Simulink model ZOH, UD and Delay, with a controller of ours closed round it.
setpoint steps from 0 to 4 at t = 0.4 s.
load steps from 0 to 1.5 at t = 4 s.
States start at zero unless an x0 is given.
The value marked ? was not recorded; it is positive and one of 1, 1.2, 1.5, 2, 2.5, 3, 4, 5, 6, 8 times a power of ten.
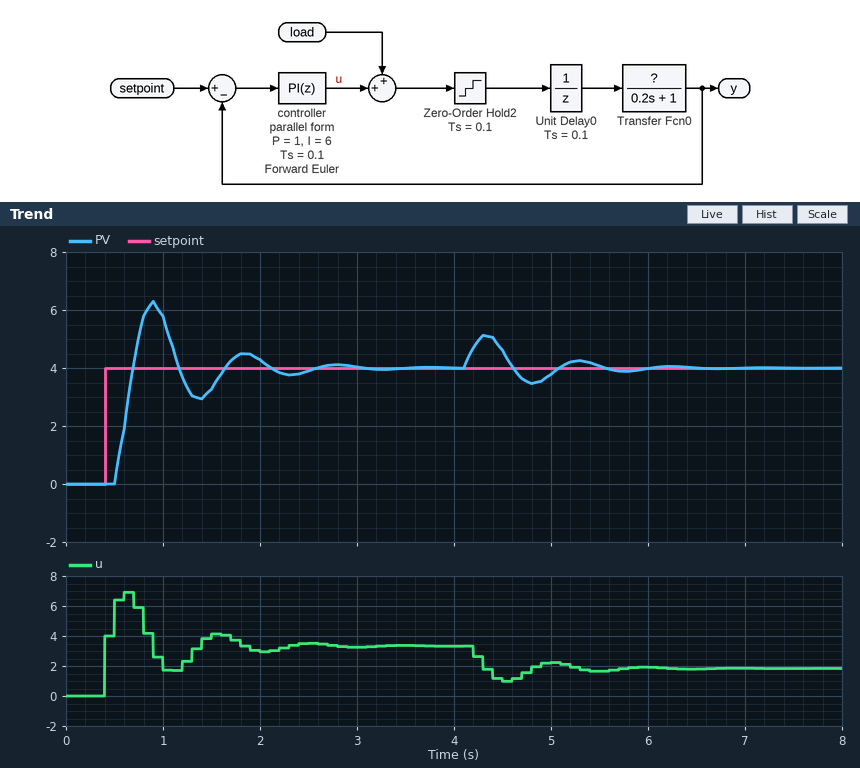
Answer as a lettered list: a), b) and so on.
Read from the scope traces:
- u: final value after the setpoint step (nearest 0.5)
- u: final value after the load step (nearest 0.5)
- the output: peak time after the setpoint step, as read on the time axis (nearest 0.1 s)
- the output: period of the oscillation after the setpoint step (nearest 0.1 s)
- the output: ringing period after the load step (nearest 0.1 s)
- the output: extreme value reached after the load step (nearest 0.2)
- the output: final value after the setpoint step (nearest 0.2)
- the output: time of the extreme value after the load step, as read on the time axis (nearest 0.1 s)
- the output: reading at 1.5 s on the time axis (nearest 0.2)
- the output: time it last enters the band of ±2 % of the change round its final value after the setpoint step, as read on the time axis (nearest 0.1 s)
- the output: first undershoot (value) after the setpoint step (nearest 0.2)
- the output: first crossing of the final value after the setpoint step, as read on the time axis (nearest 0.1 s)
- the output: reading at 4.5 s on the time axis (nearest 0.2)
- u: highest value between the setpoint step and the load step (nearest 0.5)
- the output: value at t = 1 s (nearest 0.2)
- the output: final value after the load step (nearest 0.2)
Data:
a) 3.5
b) 2.0
c) 0.9 s
d) 0.9 s
e) 1.0 s
f) 5.2
g) 4.0
h) 4.3 s
i) 3.2
j) 2.9 s
k) 3.0
l) 0.7 s
m) 4.6
n) 7.0
o) 5.8
p) 4.0
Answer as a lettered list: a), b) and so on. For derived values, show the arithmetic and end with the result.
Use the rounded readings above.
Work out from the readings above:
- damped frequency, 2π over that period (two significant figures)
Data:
a) 2π / 0.9 = 7.0 rad/s
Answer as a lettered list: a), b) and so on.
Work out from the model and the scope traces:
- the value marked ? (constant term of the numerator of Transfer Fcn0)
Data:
a) 1.2
